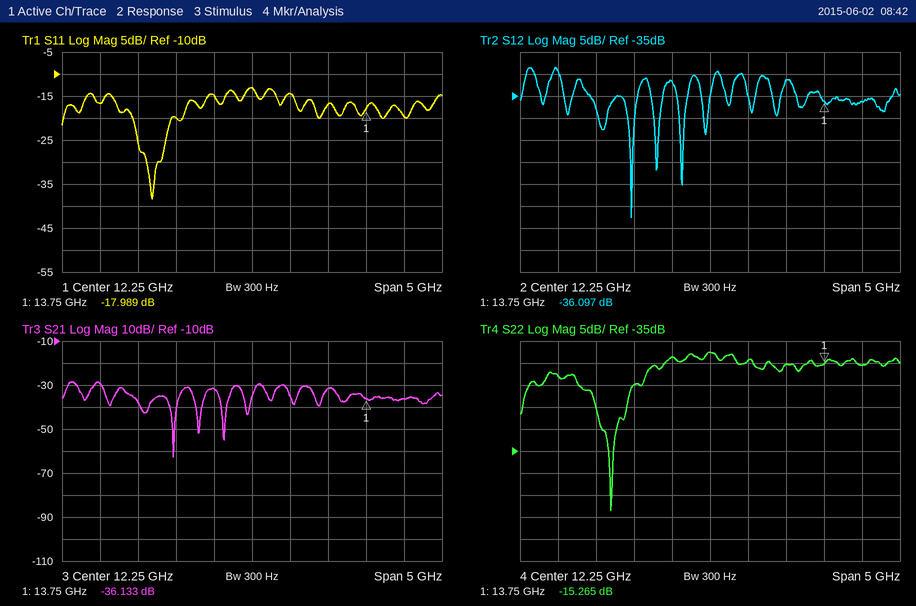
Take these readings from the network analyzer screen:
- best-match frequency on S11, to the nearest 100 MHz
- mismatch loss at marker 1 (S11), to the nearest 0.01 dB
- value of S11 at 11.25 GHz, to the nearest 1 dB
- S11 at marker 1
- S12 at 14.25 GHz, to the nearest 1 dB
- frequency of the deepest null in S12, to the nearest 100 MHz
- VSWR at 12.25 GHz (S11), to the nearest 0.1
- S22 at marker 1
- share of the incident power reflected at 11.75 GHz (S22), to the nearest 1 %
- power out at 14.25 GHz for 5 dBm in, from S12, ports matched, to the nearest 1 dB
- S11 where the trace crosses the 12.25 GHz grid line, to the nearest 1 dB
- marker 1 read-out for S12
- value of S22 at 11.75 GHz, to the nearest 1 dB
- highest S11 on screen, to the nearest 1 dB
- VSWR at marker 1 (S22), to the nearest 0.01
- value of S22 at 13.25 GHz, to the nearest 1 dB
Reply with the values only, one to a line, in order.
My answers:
10.9 GHz
0.07 dB
-20 dB
-17.989 dB
-36 dB
11.2 GHz
1.6
-15.265 dB
4 %
-31 dBm
-13 dB
-36.097 dB
-14 dB
-13 dB
1.42
-15 dB
